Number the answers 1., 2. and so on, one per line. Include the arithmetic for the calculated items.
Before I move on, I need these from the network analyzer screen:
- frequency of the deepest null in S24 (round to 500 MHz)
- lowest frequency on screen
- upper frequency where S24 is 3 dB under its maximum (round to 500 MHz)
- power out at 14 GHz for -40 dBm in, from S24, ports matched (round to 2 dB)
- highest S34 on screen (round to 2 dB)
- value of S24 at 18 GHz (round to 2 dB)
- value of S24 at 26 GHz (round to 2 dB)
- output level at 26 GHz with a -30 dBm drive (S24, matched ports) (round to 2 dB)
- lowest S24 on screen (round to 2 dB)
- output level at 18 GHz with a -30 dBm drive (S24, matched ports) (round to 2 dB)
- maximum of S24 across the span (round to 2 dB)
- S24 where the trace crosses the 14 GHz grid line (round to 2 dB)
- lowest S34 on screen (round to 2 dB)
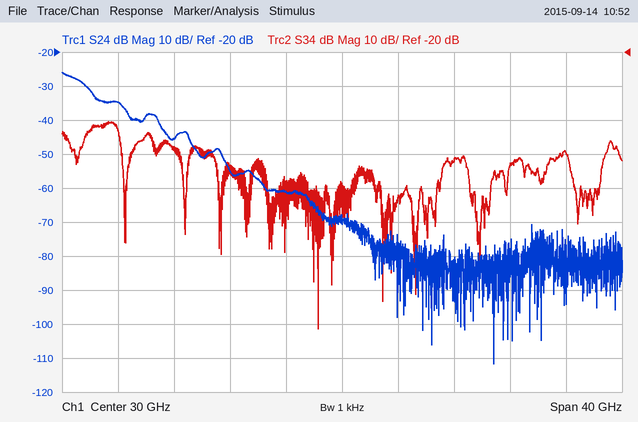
1. 41.0 GHz
2. 10 GHz
3. 11.5 GHz
4. -40 dBm + (-34 dB) = -74 dBm
5. -40 dB
6. -46 dB
7. -62 dB
8. -30 dBm + (-62 dB) = -92 dBm
9. -112 dB
10. -30 dBm + (-46 dB) = -76 dBm
11. -26 dB
12. -34 dB
13. -102 dB
